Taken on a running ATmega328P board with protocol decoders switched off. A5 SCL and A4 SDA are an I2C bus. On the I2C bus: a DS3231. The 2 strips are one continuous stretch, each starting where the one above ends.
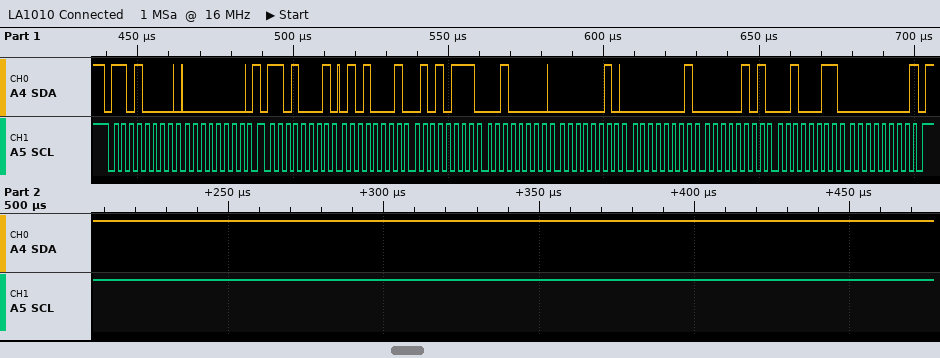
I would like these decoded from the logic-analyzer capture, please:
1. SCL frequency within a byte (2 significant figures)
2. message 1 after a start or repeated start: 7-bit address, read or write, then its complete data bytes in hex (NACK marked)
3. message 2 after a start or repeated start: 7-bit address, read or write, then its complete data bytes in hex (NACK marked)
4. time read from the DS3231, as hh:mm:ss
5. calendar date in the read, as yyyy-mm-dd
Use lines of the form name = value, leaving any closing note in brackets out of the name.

SCL frequency within a byte = 400 kHz
message 1 after a start or repeated start: 7-bit address, read or write, then its complete data bytes in hex = 0x68 write: 00
message 2 after a start or repeated start: 7-bit address, read or write, then its complete data bytes in hex = 0x68 read: 51 57 20 02 01 05 23 00 NACK
time read from the DS3231, as hh:mm:ss = 20:57:51
calendar date in the read, as yyyy-mm-dd = 2023-05-01
